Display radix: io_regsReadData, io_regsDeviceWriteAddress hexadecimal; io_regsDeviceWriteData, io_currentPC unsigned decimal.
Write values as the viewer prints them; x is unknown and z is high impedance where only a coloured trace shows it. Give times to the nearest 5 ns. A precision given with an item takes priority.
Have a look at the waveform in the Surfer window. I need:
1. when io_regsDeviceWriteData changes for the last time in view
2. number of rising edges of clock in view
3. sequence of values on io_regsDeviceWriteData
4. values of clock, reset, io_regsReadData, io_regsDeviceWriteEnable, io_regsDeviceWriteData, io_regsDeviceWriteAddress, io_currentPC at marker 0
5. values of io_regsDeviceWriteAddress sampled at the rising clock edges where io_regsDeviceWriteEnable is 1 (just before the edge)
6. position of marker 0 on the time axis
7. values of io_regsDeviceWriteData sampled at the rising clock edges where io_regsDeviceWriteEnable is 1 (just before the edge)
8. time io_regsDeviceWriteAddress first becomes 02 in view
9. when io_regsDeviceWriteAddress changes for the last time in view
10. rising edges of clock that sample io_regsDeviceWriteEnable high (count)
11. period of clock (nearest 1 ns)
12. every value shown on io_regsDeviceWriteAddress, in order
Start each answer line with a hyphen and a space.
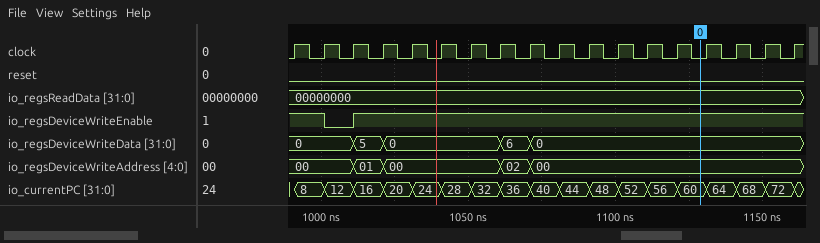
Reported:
- 1070 ns
- 18
- 0, 5, 0, 6, 0
- clock=0, reset=0, io_regsReadData=00000000, io_regsDeviceWriteEnable=1, io_regsDeviceWriteData=0, io_regsDeviceWriteAddress=00, io_currentPC=60
- 00, 00, 01, 00, 00, 00, 00, 02, 00, 00, 00, 00, 00, 00, 00, 00, 00
- 1130 ns
- 0, 0, 5, 0, 0, 0, 0, 6, 0, 0, 0, 0, 0, 0, 0, 0, 0
- 1060 ns
- 1070 ns
- 17
- 10 ns
- 00, 01, 00, 02, 00
